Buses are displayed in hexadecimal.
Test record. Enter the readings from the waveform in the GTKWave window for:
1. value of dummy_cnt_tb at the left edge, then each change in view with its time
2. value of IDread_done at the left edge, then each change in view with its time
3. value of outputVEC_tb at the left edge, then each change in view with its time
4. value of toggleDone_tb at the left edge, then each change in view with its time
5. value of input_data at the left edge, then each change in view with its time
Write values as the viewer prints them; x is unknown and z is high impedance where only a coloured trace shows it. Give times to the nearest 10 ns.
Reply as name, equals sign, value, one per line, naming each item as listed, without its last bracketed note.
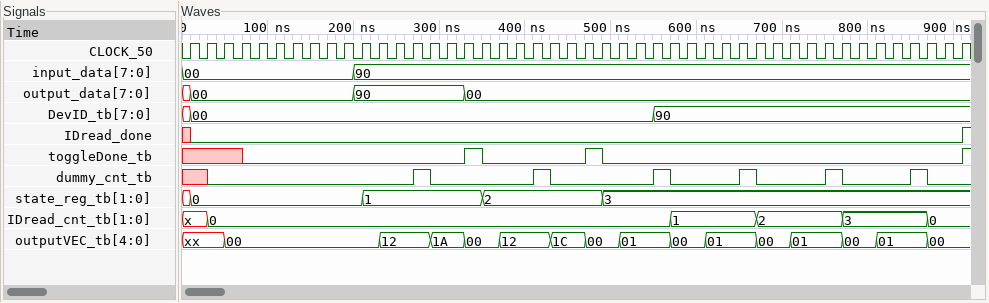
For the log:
value of dummy_cnt_tb at the left edge, then each change in view with its time = x, 0 at 30 ns, 1 at 270 ns, 0 at 290 ns, 1 at 410 ns, 0 at 430 ns, 1 at 550 ns, 0 at 570 ns, 1 at 650 ns, 0 at 670 ns, 1 at 750 ns, 0 at 770 ns, 1 at 850 ns, 0 at 870 ns
value of IDread_done at the left edge, then each change in view with its time = x, 0 at 10 ns, 1 at 910 ns
value of outputVEC_tb at the left edge, then each change in view with its time = xx, 00 at 50 ns, 12 at 230 ns, 1A at 290 ns, 00 at 330 ns, 12 at 370 ns, 1C at 430 ns, 00 at 470 ns, 01 at 510 ns, 00 at 570 ns, 01 at 610 ns, 00 at 670 ns, 01 at 710 ns, 00 at 770 ns, 01 at 810 ns, 00 at 870 ns
value of toggleDone_tb at the left edge, then each change in view with its time = x, 0 at 70 ns, 1 at 330 ns, 0 at 350 ns, 1 at 470 ns, 0 at 490 ns, 1 at 910 ns
value of input_data at the left edge, then each change in view with its time = 00, 90 at 200 ns
